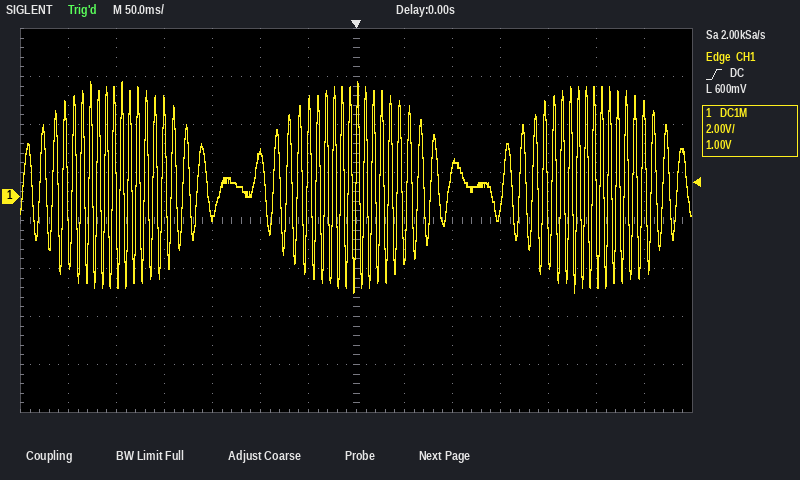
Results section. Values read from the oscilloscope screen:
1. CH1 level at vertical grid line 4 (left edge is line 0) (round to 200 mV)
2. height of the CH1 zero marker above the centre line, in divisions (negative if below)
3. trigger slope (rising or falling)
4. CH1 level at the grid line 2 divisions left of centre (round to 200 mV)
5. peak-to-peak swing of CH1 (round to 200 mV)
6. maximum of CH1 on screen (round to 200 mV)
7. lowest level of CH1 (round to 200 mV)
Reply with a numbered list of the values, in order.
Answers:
1. -800 mV
2. +0.5 div
3. rising
4. 1.8 V
5. 8.8 V
6. 4.8 V
7. -4.0 V
